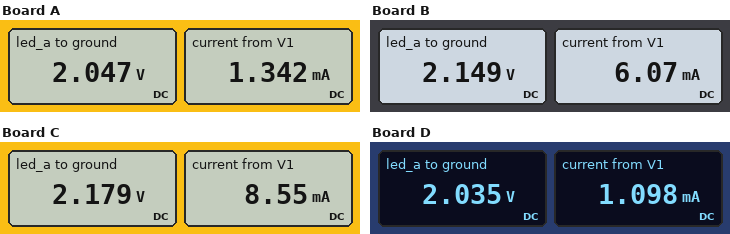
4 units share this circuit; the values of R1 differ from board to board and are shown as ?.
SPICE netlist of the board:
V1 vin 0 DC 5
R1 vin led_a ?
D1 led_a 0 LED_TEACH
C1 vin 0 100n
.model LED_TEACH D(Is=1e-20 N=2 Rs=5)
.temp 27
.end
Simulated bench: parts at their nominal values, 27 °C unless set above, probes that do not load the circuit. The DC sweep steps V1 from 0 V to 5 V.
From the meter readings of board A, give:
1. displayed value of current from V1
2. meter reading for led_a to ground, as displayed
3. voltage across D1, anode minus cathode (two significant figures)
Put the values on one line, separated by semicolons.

1.342 mA; 2.047 V; 2.0 V
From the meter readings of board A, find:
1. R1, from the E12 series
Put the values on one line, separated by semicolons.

2.2 kΩ
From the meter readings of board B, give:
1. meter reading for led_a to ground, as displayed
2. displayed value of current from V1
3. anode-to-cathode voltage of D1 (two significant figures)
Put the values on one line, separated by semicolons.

2.149 V; 6.07 mA; 2.1 V
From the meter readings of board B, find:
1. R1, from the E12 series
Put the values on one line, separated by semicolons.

470 Ω
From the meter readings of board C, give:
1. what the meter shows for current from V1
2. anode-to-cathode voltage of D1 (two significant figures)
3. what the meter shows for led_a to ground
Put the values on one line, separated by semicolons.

8.55 mA; 2.2 V; 2.179 V
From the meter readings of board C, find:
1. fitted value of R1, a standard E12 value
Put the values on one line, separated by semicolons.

330 Ω
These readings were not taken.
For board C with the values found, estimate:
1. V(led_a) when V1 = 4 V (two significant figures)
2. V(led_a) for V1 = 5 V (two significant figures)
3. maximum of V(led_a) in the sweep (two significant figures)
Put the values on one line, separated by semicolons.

2.1 V; 2.2 V; 2.2 V
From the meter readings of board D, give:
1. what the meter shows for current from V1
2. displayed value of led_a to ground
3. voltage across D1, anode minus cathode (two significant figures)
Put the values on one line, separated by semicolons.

1.098 mA; 2.035 V; 2.0 V
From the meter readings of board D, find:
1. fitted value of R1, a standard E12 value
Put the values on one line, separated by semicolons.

2.7 kΩ
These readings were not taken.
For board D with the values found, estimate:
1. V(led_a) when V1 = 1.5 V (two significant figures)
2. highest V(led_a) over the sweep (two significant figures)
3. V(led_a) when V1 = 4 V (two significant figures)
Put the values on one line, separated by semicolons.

1.5 V; 2.0 V; 2.0 V
